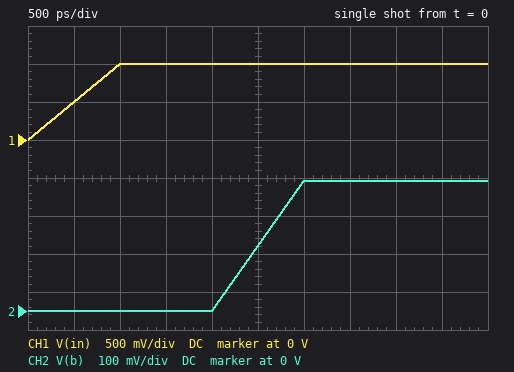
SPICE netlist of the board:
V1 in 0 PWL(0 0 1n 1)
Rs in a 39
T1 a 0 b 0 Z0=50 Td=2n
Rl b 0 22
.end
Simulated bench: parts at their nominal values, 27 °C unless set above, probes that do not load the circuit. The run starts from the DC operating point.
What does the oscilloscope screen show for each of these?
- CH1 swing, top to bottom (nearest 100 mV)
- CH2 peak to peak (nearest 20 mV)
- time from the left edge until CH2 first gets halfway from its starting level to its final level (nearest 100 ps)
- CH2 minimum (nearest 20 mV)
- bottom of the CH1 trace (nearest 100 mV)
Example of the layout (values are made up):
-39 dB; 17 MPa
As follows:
1.0 V; 340 mV; 2.5 ns; 0 V; 0 V
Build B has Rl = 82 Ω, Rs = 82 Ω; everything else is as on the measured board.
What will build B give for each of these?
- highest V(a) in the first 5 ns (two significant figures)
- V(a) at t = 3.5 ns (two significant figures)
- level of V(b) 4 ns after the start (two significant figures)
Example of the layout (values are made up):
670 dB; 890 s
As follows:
490 mV; 380 mV; 470 mV
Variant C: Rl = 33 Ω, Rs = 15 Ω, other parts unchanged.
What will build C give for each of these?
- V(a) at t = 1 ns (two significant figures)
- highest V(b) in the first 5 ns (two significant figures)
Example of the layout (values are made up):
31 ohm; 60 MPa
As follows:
770 mV; 610 mV
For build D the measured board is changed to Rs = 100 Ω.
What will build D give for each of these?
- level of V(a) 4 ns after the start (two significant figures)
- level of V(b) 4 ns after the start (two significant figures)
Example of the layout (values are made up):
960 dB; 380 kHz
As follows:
330 mV; 200 mV
